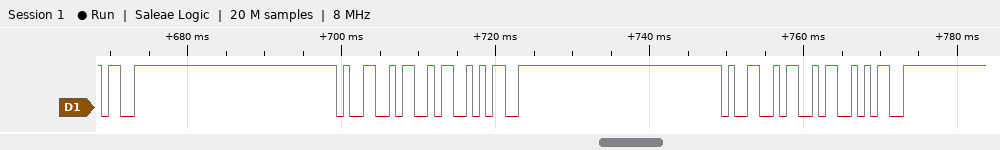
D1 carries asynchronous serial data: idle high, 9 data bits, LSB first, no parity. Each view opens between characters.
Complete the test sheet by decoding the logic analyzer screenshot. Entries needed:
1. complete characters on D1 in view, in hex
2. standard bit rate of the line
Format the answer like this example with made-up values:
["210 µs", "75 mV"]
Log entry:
["1F3, 99, 9A, 1F3, 99, 9A, 1F3", "1200 baud"]
